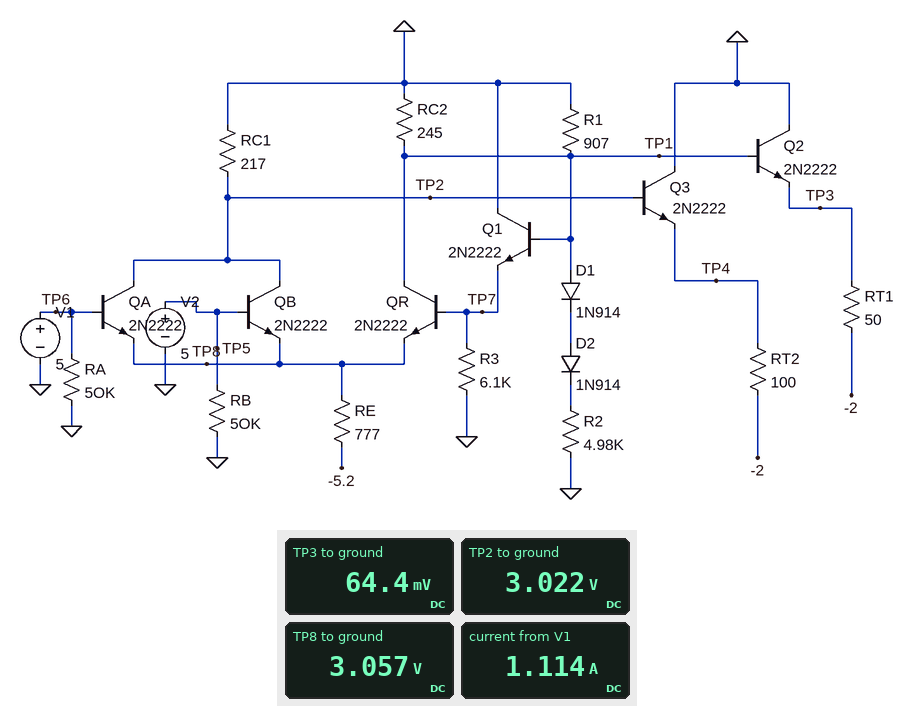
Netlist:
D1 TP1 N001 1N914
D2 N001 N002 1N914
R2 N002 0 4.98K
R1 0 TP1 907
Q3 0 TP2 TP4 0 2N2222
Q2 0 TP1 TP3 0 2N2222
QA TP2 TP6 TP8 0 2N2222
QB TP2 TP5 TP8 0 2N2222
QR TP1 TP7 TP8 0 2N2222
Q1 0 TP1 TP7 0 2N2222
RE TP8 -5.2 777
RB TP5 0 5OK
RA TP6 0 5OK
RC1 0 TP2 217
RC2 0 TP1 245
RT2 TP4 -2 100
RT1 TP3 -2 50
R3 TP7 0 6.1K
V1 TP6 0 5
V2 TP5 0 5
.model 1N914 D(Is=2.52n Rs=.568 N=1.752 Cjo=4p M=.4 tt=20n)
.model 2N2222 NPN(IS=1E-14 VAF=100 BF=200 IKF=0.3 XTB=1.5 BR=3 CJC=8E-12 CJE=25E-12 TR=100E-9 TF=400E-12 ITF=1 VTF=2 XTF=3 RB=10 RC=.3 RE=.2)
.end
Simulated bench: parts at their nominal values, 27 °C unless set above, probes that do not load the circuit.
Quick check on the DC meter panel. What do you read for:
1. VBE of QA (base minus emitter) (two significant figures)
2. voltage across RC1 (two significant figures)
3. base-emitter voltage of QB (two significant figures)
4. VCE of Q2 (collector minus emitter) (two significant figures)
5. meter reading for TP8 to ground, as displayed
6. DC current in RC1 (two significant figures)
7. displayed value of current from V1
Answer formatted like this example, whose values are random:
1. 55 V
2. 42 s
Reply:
1. 1.9 V
2. 3.0 V
3. 1.9 V
4. -64 mV
5. 3.057 V
6. 14 mA
7. 1.114 A
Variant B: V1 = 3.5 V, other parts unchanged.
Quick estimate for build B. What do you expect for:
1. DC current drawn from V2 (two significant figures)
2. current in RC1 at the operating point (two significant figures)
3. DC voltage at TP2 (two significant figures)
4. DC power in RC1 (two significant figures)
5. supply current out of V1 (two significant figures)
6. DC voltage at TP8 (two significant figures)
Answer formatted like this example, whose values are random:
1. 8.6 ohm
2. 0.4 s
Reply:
1. 1.2 A
2. 12 mA
3. 2.5 V
4. 30 mW
5. 720 mA
6. 2.6 V
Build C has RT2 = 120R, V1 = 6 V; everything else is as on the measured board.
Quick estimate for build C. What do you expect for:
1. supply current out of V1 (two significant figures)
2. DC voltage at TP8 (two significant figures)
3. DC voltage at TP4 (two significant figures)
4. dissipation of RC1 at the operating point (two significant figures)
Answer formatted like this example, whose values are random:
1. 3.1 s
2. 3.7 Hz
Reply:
1. 1.4 A
2. 3.4 V
3. 74 mV
4. 52 mW
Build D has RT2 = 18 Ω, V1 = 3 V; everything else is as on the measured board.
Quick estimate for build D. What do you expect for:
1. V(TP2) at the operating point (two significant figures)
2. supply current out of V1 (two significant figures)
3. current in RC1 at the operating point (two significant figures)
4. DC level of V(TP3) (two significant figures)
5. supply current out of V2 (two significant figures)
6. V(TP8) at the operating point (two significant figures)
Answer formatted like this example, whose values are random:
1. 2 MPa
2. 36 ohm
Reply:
1. 2.4 V
2. 600 mA
3. 11 mA
4. 48 mV
5. 1.2 A
6. 2.5 V
